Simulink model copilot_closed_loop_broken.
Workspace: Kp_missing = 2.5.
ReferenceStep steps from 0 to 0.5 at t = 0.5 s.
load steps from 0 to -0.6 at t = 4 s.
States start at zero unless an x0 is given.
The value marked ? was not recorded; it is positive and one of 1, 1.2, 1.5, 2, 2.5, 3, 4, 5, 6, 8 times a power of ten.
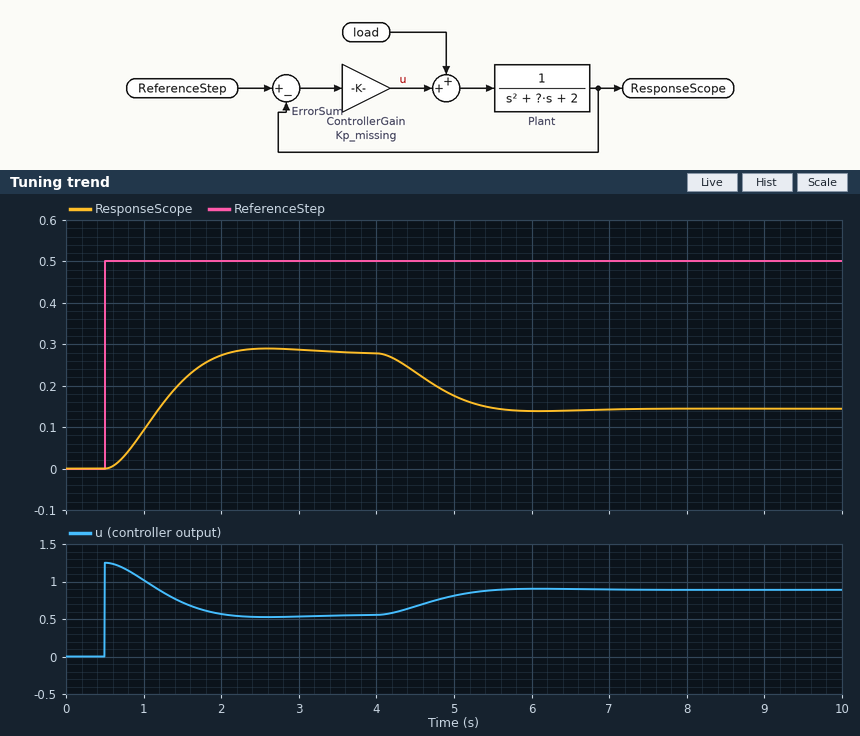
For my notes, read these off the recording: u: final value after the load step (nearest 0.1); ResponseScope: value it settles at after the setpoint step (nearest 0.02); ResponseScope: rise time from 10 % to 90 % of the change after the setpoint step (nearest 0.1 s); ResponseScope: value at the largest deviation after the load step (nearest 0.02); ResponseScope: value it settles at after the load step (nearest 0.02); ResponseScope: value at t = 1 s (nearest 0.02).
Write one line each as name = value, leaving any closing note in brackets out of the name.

u: final value after the load step = 0.9
ResponseScope: value it settles at after the setpoint step = 0.28
ResponseScope: rise time from 10 % to 90 % of the change after the setpoint step = 1.0 s
ResponseScope: value at the largest deviation after the load step = 0.14
ResponseScope: value it settles at after the load step = 0.14
ResponseScope: value at t = 1 s = 0.10
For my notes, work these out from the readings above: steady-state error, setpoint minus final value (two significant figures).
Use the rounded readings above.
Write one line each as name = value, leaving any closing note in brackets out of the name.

steady-state error, setpoint minus final value = 0.22
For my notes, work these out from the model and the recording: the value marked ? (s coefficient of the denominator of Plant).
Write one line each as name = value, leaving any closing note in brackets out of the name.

the value marked ? = 3
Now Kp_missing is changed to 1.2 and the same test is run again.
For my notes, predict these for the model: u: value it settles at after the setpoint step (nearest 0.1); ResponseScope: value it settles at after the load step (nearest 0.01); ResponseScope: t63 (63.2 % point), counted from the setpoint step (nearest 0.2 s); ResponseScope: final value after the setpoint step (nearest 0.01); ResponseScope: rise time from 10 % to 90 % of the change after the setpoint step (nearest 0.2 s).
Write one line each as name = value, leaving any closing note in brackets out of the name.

u: value it settles at after the setpoint step = 0.4
ResponseScope: value it settles at after the load step = 0.00
ResponseScope: t63 (63.2 % point), counted from the setpoint step = 1.0 s
ResponseScope: final value after the setpoint step = 0.19
ResponseScope: rise time from 10 % to 90 % of the change after the setpoint step = 1.4 s
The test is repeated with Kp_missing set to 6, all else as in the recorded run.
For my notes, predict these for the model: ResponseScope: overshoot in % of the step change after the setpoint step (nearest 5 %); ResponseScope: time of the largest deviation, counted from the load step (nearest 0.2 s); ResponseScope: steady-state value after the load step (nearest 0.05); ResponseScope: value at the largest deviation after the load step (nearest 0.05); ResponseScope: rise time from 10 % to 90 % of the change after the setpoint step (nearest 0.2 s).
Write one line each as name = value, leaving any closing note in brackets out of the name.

ResponseScope: overshoot in % of the step change after the setpoint step = 15 %
ResponseScope: time of the largest deviation, counted from the load step = 1.4 s
ResponseScope: steady-state value after the load step = 0.30
ResponseScope: value at the largest deviation after the load step = 0.30
ResponseScope: rise time from 10 % to 90 % of the change after the setpoint step = 0.6 s
